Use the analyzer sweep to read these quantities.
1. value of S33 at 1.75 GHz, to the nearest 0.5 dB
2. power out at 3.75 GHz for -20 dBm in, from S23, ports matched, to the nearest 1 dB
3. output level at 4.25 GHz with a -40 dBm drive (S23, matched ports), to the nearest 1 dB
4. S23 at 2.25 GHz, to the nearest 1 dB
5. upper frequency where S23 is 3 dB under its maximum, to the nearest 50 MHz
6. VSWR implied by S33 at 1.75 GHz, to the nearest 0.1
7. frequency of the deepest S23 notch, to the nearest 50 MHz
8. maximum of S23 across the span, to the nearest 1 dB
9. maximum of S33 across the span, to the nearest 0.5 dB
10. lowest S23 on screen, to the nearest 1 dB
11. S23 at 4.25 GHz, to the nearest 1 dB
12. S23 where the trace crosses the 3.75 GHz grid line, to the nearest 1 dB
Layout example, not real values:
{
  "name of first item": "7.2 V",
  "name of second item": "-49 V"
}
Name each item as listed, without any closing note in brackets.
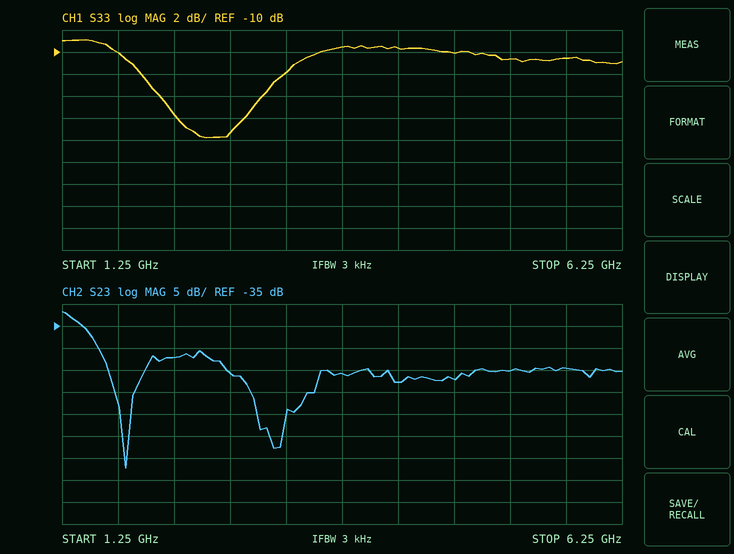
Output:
{
  "value of S33 at 1.75 GHz, to the nearest 0.5 dB": "-10.0 dB",
  "power out at 3.75 GHz for -20 dBm in, from S23, ports matched, to the nearest 1 dB": "-66 dBm",
  "output level at 4.25 GHz with a -40 dBm drive (S23, matched ports), to the nearest 1 dB": "-88 dBm",
  "S23 at 2.25 GHz, to the nearest 1 dB": "-42 dB",
  "upper frequency where S23 is 3 dB under its maximum, to the nearest 50 MHz": "1.40 GHz",
  "VSWR implied by S33 at 1.75 GHz, to the nearest 0.1": "1.9",
  "frequency of the deepest S23 notch, to the nearest 50 MHz": "1.80 GHz",
  "maximum of S23 across the span, to the nearest 1 dB": "-32 dB",
  "maximum of S33 across the span, to the nearest 0.5 dB": "-9.0 dB",
  "lowest S23 on screen, to the nearest 1 dB": "-67 dB",
  "S23 at 4.25 GHz, to the nearest 1 dB": "-48 dB",
  "S23 where the trace crosses the 3.75 GHz grid line, to the nearest 1 dB": "-46 dB"
}
